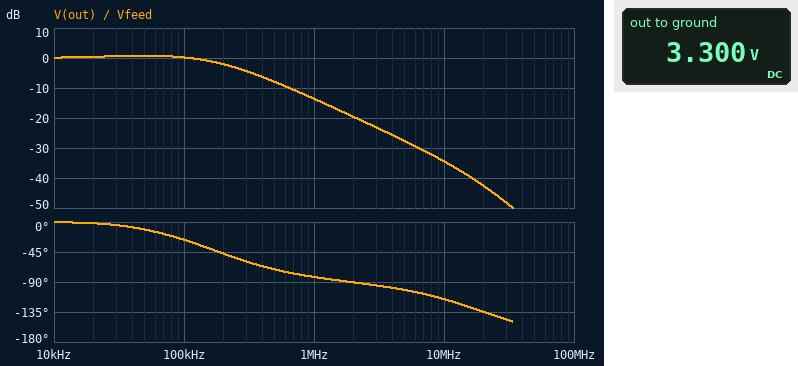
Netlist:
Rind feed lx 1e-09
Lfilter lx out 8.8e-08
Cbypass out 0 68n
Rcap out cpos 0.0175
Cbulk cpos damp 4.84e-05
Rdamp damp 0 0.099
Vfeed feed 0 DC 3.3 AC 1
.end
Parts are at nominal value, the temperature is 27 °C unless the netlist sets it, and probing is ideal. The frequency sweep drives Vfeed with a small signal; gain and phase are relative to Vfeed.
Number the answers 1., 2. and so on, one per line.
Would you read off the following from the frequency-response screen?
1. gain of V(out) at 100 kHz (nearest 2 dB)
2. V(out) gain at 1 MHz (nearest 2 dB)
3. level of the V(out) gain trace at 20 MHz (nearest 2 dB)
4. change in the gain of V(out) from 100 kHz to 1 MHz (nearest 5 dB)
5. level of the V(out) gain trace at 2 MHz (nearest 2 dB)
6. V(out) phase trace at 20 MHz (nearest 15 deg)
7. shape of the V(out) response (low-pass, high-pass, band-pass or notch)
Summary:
1. 0 dB
2. -14 dB
3. -42 dB
4. -15 dB
5. -20 dB
6. -135 deg
7. low-pass
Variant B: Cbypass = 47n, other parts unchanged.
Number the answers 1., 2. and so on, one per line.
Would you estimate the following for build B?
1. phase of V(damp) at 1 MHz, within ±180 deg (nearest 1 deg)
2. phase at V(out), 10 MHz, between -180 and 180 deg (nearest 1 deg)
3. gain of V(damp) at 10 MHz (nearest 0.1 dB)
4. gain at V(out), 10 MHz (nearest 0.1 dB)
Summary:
1. -80 deg
2. -108 deg
3. -35.4 dB
4. -34.0 dB
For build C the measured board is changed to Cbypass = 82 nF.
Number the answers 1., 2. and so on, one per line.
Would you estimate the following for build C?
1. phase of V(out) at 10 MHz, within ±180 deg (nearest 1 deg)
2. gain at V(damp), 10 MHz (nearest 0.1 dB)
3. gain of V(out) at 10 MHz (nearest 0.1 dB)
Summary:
1. -120 deg
2. -36.2 dB
3. -34.8 dB
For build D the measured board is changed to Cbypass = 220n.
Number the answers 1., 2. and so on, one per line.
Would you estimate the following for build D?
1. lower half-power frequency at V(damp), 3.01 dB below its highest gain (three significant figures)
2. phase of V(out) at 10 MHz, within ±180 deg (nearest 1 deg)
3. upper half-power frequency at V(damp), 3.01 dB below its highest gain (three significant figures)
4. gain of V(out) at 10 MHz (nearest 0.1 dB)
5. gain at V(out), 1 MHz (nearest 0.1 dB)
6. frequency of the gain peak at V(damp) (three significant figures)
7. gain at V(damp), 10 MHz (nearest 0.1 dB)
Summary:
1. 25.4 kHz
2. -148 deg
3. 241 kHz
4. -39.0 dB
5. -13.5 dB
6. 78.3 kHz
7. -40.4 dB
